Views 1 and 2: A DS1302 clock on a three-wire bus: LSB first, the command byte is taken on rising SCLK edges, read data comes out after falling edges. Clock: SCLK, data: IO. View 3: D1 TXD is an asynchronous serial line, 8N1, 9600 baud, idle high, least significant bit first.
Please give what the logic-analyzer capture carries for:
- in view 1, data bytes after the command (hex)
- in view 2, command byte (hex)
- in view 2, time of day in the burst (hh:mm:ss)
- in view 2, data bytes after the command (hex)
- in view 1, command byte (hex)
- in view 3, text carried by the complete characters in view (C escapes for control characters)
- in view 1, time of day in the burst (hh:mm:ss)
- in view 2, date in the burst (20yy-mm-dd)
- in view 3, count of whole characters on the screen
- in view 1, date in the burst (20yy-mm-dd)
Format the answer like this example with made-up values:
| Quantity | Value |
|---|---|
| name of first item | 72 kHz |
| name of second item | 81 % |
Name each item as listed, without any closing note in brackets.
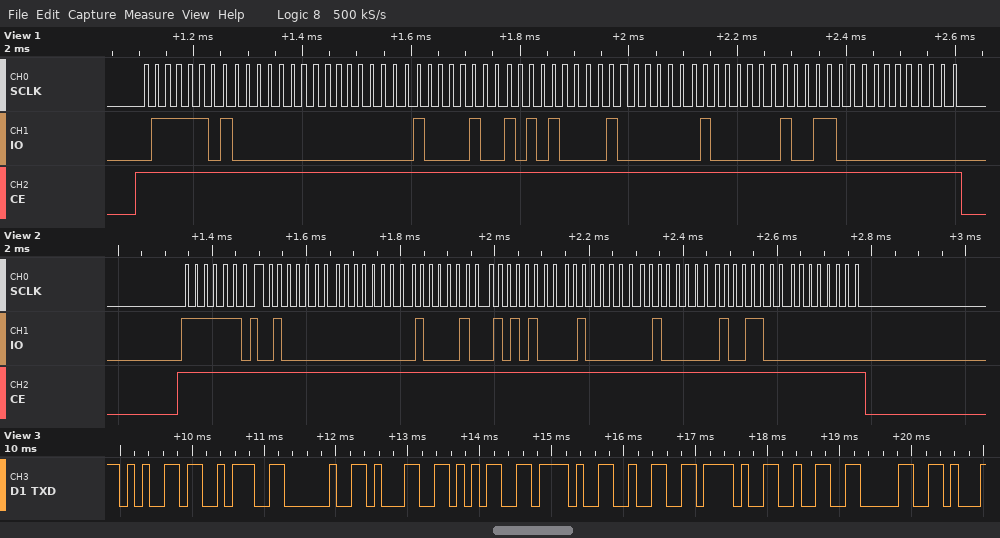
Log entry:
| Quantity | Value |
|---|---|
| in view 1, data bytes after the command | 00 00 21 15 02 02 19 00 |
| in view 2, command byte | 0xBF |
| in view 2, time of day in the burst | 21:00:02 |
| in view 2, data bytes after the command | 02 00 21 15 02 02 19 00 |
| in view 1, command byte | 0xBE |
| in view 3, text carried by the complete characters in view | "e: 15/2/20" |
| in view 1, time of day in the burst | 21:00:00 |
| in view 2, date in the burst | 2019-02-15 |
| in view 3, count of whole characters on the screen | 10 |
| in view 1, date in the burst | 2019-02-15 |
